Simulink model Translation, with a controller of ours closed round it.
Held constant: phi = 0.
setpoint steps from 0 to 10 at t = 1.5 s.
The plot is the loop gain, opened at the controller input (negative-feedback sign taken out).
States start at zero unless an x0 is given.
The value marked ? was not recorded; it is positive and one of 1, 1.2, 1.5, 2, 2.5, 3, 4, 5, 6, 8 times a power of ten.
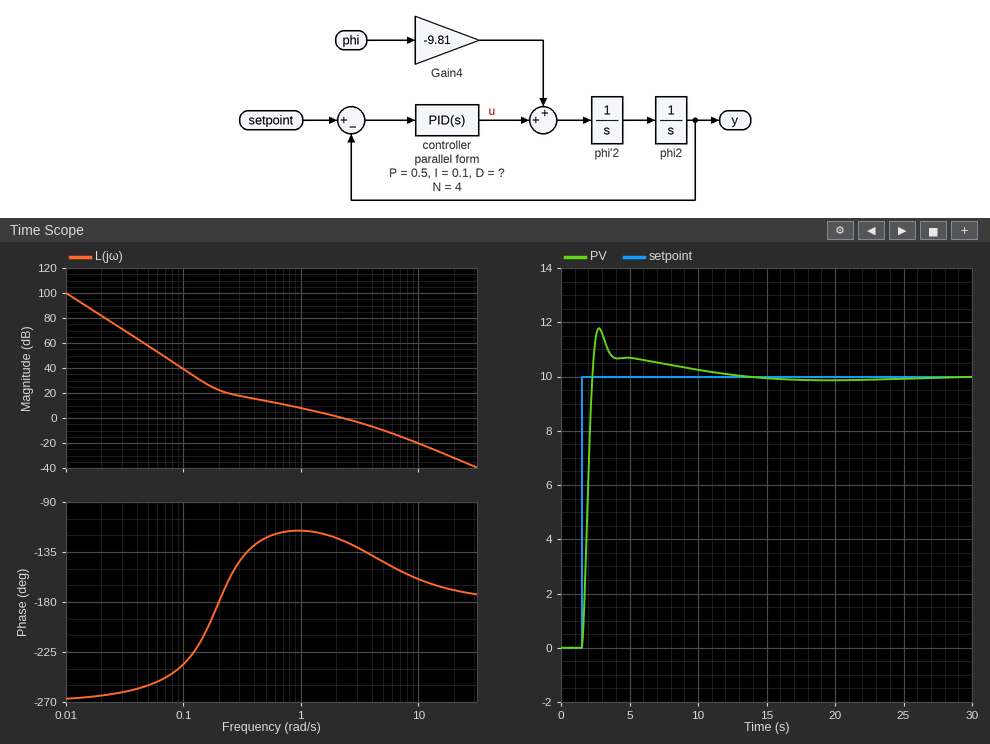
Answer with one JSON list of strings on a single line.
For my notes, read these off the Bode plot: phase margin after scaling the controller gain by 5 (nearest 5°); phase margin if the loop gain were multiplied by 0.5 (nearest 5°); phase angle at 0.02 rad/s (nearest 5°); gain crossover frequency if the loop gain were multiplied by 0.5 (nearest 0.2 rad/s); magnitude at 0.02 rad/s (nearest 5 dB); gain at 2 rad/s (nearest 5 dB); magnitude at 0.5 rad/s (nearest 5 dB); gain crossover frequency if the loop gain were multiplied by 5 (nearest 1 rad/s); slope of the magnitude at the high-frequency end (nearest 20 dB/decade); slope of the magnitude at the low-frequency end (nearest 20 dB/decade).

["30°", "65°", "-265°", "1.2 rad/s", "80 dB", "0 dB", "15 dB", "7 rad/s", "-40 dB/decade", "-60 dB/decade"]
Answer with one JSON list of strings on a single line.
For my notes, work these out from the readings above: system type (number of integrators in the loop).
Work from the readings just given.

["3"]
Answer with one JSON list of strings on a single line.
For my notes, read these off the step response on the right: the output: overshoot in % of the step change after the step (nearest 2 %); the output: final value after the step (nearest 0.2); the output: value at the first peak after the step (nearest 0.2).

["18 %", "10.0", "11.8"]
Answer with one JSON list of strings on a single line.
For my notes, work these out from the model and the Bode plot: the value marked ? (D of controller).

["2.5"]
